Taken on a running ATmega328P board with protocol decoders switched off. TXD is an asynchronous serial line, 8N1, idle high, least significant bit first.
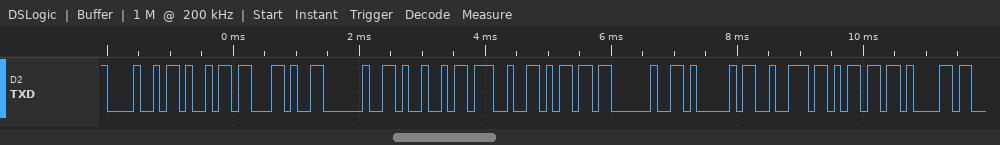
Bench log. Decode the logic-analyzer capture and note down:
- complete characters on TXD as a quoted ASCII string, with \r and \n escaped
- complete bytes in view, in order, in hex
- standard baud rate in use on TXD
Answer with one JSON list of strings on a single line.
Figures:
["\"Hi, I'm Arma\"", "0x48 0x69 0x2C 0x20 0x49 0x27 0x6D 0x20 0x41 0x72 0x6D 0x61", "9600 baud"]
